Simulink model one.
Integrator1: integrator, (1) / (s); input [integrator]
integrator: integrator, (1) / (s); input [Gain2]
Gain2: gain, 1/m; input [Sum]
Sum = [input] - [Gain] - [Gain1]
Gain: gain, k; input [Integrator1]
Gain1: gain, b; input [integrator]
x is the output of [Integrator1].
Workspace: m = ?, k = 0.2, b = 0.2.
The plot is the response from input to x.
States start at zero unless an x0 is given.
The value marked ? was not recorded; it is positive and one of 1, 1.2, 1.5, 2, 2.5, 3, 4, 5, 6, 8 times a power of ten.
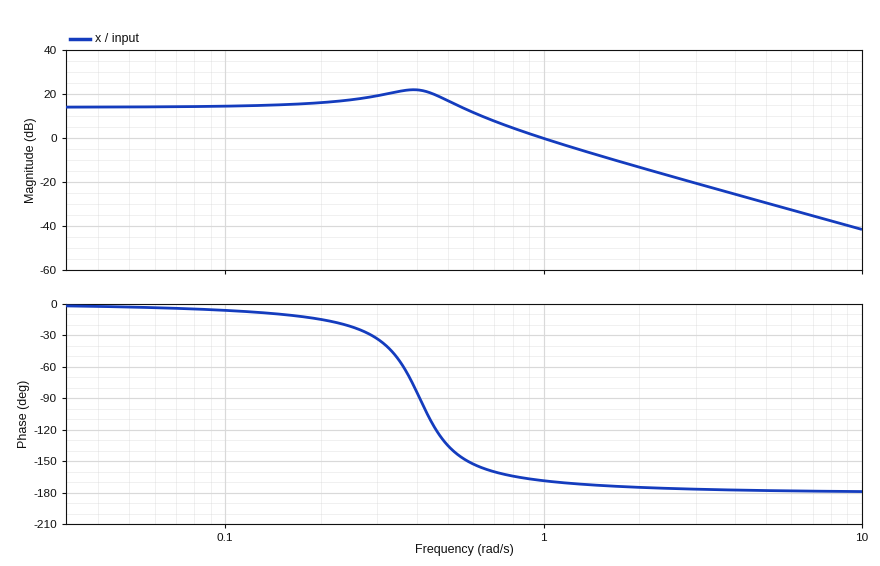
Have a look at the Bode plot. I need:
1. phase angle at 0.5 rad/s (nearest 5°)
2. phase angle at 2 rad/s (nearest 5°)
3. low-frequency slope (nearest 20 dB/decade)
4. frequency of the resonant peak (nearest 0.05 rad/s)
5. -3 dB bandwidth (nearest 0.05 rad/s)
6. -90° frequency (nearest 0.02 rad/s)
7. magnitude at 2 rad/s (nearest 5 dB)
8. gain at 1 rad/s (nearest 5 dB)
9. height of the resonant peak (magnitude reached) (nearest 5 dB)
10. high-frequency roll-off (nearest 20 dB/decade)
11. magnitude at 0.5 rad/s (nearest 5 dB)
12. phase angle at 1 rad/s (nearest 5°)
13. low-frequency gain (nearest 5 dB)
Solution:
-135°
-175°
0 dB/decade
0.40 rad/s
0.60 rad/s
0.40 rad/s
-15 dB
0 dB
20 dB
-40 dB/decade
15 dB
-170°
15 dB
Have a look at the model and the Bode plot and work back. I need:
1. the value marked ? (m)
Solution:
1.2
